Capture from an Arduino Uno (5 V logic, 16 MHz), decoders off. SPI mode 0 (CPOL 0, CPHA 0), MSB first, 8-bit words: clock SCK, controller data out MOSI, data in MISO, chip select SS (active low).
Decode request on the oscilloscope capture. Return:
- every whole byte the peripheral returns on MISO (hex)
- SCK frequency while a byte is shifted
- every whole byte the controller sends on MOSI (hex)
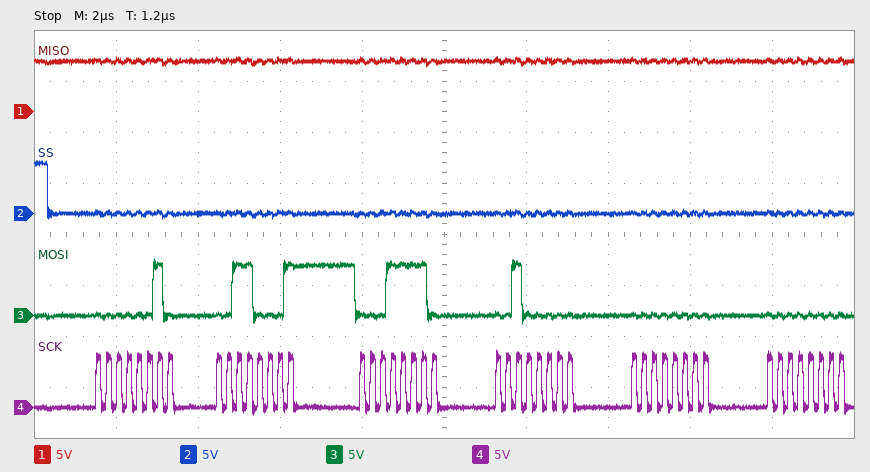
FF FF FF FF FF FF
4 MHz
02 31 1E 20 00 00
